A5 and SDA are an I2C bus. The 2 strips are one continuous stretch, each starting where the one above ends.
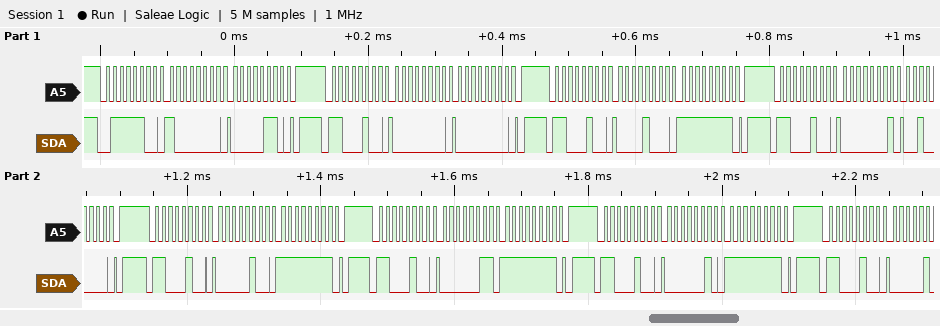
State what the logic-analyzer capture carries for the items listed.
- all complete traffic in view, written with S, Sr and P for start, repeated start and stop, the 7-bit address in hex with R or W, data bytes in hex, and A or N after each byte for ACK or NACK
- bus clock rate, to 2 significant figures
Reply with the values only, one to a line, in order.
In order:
S 3EW A 80 A 06 A P S 62W A 00 A 00 A P S 62W A 08 A FF A P S 62W A 01 A 20 A P S 62W A 04 A FF A P S 62W A 03 A FF A P S 62W A 02 A FF A P S 62W A
100 kHz
